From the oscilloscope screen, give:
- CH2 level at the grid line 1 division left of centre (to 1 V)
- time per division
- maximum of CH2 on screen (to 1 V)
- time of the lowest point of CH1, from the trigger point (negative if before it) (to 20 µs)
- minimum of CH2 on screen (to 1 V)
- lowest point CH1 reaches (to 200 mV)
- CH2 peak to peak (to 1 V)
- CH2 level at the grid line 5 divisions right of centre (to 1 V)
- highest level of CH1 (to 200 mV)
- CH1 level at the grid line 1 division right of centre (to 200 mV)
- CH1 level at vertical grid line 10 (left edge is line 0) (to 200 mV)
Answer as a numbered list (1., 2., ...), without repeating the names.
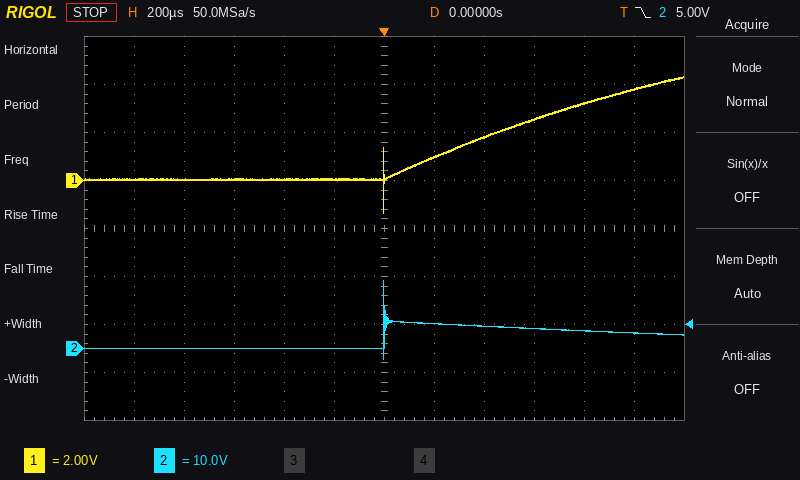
1. 0 V
2. 200 µs
3. 14 V
4. 0 µs
5. -2 V
6. -1.4 V
7. 16 V
8. 3 V
9. 4.4 V
10. 1.0 V
11. 3.2 V
